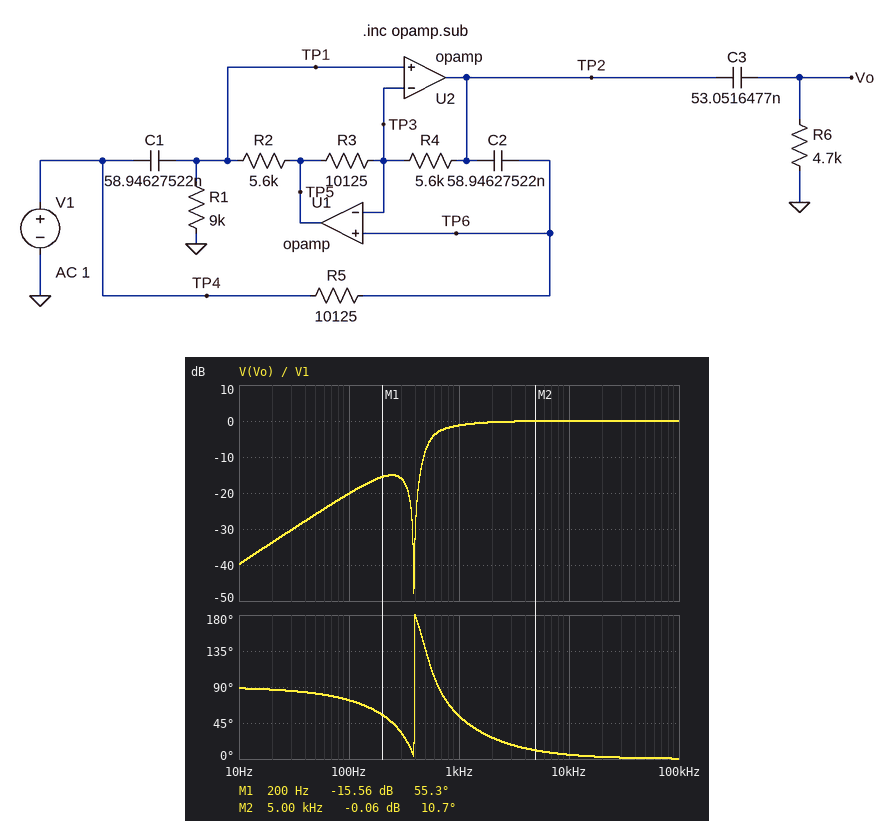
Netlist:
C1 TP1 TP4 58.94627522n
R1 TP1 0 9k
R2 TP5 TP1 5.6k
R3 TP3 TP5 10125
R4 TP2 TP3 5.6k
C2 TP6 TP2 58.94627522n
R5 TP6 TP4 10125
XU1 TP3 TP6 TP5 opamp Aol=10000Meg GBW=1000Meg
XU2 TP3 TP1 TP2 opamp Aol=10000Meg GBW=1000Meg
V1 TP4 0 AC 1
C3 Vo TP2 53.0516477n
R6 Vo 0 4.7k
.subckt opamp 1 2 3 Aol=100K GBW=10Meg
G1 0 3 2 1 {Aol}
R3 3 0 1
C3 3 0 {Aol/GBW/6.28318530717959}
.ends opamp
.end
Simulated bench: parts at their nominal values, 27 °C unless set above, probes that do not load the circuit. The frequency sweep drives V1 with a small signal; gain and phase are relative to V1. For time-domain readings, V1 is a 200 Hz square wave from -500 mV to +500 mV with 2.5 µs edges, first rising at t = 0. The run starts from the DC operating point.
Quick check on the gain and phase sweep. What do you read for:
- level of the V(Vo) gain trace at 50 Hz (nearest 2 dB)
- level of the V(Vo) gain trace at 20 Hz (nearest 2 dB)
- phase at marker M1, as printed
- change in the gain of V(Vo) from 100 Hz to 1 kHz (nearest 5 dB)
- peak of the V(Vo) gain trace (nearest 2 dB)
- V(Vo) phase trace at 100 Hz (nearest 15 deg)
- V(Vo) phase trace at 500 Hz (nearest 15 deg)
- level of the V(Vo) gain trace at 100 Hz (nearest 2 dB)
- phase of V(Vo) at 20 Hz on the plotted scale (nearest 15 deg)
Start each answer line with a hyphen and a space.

- -26 dB
- -34 dB
- 55.3 deg
- 20 dB
- 0 dB
- 75 deg
- 135 deg
- -20 dB
- 90 deg
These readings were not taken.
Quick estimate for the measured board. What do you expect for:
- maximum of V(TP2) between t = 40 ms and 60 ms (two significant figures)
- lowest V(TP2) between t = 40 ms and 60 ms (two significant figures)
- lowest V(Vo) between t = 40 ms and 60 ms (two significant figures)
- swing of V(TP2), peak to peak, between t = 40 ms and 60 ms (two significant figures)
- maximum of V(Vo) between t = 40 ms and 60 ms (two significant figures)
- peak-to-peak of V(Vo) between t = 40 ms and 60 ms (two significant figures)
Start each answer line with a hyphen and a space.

- 690 mV
- -690 mV
- -1.0 V
- 1.4 V
- 1.0 V
- 2.1 V
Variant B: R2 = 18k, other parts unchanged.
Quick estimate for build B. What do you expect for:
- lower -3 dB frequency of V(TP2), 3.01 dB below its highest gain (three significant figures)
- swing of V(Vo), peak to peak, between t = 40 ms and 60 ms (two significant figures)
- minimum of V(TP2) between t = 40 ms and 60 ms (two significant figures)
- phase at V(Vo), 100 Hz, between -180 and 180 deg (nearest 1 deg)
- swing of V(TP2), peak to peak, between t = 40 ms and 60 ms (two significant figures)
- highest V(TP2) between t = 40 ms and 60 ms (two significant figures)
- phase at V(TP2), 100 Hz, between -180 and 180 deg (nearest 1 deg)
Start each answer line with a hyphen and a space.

- 220 Hz
- 1.9 V
- -1.1 V
- -125 deg
- 2.3 V
- 1.1 V
- 154 deg
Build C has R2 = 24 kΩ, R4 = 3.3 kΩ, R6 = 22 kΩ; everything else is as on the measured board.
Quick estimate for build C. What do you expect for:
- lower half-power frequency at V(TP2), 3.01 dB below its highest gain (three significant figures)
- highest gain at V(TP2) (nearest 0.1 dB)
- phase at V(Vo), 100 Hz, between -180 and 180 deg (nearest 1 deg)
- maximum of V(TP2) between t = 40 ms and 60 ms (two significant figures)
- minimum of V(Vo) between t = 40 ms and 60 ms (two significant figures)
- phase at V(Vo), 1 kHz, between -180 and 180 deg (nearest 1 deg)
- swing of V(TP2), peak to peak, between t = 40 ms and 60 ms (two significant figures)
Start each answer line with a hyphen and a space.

- 279 Hz
- 0.8 dB
- 34 deg
- 920 mV
- -880 mV
- 26 deg
- 1.8 V
